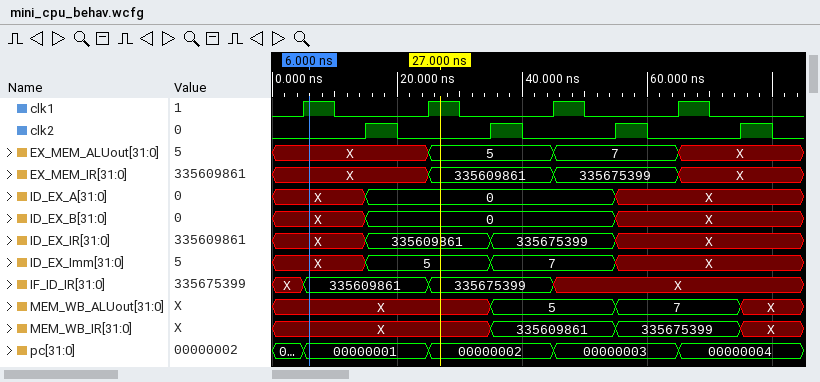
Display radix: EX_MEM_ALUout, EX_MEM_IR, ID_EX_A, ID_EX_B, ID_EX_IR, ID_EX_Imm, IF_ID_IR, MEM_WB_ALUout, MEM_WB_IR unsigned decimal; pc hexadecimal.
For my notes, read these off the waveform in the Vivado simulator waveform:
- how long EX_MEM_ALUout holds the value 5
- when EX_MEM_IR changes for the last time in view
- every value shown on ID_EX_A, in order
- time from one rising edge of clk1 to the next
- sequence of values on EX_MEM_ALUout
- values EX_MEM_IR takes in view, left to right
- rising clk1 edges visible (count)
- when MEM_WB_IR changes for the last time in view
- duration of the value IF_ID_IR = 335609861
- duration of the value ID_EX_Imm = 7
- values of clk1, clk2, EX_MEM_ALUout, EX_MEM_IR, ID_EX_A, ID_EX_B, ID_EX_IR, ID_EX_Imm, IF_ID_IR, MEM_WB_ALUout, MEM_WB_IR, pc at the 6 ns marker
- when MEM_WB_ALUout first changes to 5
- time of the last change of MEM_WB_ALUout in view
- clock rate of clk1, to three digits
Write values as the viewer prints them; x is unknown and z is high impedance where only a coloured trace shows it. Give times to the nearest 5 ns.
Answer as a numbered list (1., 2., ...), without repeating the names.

1. 20 ns
2. 65 ns
3. X, 0, X
4. 20 ns
5. X, 5, 7, X
6. X, 335609861, 335675399, X
7. 4
8. 75 ns
9. 20 ns
10. 20 ns
11. clk1=1, clk2=0, EX_MEM_ALUout=X, EX_MEM_IR=X, ID_EX_A=X, ID_EX_B=X, ID_EX_IR=X, ID_EX_Imm=X, IF_ID_IR=335609861, MEM_WB_ALUout=X, MEM_WB_IR=X, pc=00000001
12. 35 ns
13. 75 ns
14. 50.0 MHz
